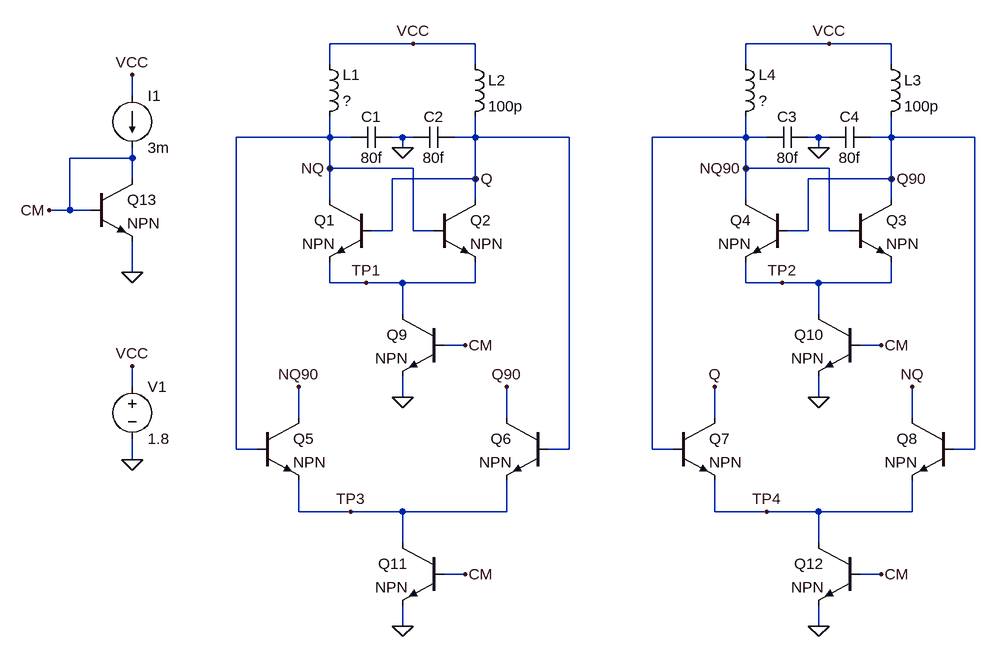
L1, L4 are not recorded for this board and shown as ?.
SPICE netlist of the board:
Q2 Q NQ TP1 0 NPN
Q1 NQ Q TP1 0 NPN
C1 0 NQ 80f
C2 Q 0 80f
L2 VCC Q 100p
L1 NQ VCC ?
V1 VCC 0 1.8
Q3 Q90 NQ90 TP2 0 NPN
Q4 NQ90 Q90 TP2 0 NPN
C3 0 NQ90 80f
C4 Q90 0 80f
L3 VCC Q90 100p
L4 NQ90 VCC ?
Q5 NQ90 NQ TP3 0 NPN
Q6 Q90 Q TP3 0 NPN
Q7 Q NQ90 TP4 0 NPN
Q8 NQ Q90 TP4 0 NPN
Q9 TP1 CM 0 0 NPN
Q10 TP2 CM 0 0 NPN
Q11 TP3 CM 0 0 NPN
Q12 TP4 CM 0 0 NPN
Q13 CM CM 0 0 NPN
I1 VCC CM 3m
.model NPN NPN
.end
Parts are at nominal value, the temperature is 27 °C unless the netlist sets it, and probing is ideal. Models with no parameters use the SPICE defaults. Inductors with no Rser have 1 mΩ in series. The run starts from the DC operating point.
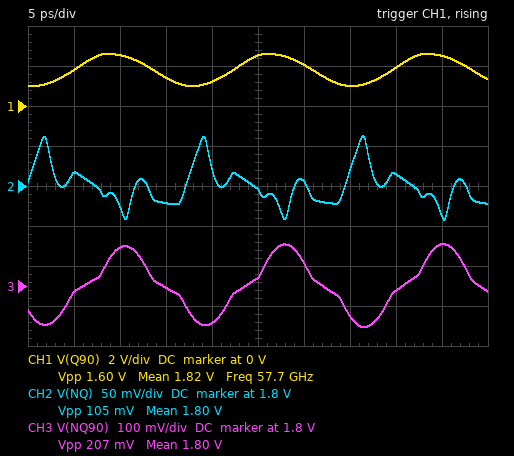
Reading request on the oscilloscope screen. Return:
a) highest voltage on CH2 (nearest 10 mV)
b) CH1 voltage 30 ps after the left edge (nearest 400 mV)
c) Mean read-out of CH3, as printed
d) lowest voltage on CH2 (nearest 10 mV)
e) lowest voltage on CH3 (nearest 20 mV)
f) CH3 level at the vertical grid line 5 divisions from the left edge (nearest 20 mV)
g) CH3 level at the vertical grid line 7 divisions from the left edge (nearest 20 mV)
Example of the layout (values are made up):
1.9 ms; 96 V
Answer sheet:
1.86 V; 2.0 V; 1.80 V; 1.76 V; 1.70 V; 1.82 V; 1.72 V
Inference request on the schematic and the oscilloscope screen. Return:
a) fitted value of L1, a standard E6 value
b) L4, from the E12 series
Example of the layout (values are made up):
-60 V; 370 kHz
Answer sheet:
220 pH; 56 pH
